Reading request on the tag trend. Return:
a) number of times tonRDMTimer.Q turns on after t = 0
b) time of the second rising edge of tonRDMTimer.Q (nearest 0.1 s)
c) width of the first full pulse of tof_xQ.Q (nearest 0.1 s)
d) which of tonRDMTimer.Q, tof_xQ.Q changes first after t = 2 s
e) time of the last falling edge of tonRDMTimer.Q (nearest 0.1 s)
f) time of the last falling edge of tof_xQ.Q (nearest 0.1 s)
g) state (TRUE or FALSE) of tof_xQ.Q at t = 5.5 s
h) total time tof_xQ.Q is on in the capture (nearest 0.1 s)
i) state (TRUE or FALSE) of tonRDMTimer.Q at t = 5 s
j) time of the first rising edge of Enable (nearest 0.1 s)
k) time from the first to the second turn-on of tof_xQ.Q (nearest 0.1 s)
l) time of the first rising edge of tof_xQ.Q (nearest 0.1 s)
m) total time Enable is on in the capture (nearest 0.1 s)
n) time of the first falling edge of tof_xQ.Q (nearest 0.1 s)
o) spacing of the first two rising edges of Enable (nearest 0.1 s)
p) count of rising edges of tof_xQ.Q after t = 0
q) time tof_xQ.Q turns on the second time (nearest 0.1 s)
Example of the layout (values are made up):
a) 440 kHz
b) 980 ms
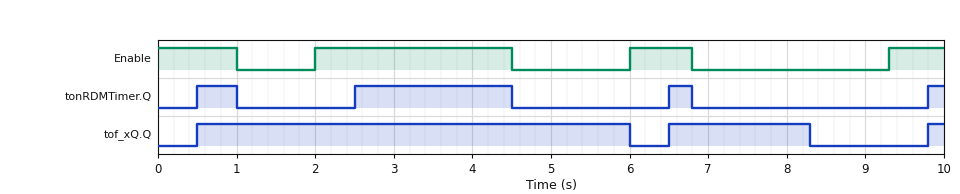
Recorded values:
a) 4
b) 2.5 s
c) 5.5 s
d) tonRDMTimer.Q
e) 6.8 s
f) 8.3 s
g) TRUE
h) 7.5 s
i) FALSE
j) 2.0 s
k) 6.0 s
l) 0.5 s
m) 5.0 s
n) 6.0 s
o) 4.0 s
p) 3
q) 6.5 s
